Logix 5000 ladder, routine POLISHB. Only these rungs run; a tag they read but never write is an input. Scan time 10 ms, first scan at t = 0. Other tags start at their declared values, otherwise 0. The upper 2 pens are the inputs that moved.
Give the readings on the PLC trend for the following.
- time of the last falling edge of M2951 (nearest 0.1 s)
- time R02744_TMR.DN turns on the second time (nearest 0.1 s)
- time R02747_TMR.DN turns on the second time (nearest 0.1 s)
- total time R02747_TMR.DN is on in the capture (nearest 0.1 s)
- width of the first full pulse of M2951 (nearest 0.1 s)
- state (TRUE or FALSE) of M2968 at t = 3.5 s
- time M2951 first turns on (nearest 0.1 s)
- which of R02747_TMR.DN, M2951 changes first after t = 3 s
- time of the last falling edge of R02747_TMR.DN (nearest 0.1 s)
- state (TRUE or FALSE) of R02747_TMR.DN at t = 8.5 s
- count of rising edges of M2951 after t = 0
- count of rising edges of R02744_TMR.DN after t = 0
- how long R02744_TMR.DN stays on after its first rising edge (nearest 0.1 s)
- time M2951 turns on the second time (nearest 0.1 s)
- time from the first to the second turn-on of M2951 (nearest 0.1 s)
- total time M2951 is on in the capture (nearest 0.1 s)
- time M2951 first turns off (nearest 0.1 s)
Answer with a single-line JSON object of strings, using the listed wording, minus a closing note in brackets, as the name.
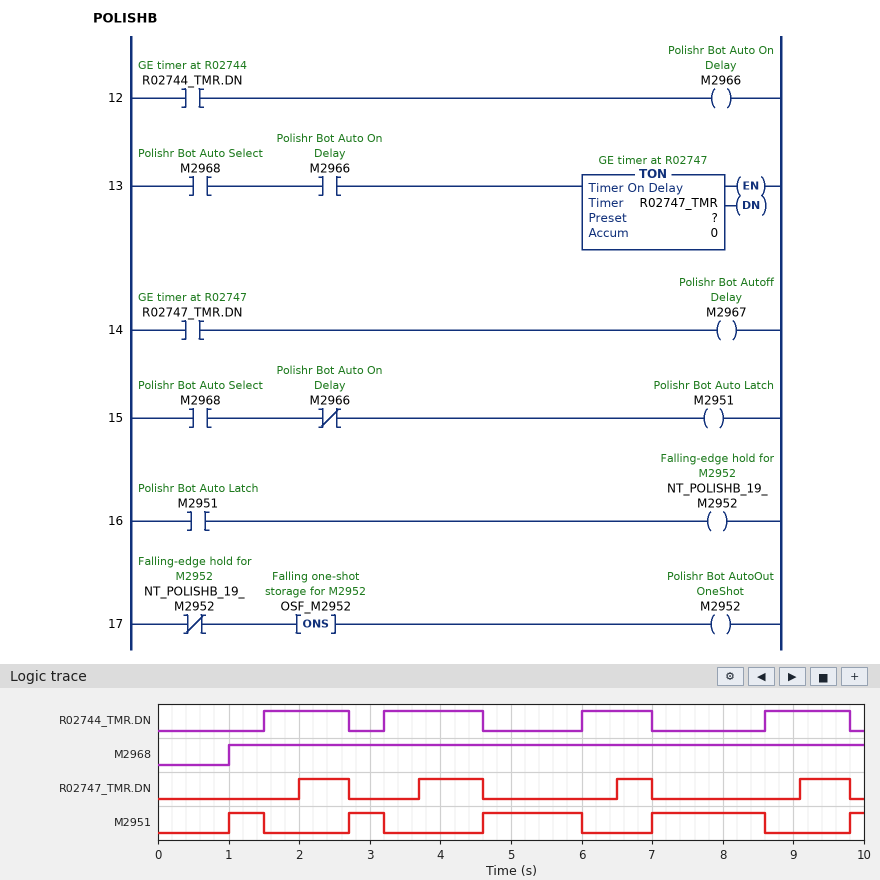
{"time of the last falling edge of M2951": "8.6 s", "time R02744_TMR.DN turns on the second time": "3.2 s", "time R02747_TMR.DN turns on the second time": "3.7 s", "total time R02747_TMR.DN is on in the capture": "2.8 s", "width of the first full pulse of M2951": "0.5 s", "state (TRUE or FALSE) of M2968 at t = 3.5 s": "TRUE", "time M2951 first turns on": "1.0 s", "which of R02747_TMR.DN, M2951 changes first after t = 3 s": "M2951", "time of the last falling edge of R02747_TMR.DN": "9.8 s", "state (TRUE or FALSE) of R02747_TMR.DN at t = 8.5 s": "FALSE", "count of rising edges of M2951 after t = 0": "5", "count of rising edges of R02744_TMR.DN after t = 0": "4", "how long R02744_TMR.DN stays on after its first rising edge": "1.2 s", "time M2951 turns on the second time": "2.7 s", "time from the first to the second turn-on of M2951": "1.7 s", "total time M2951 is on in the capture": "4.2 s", "time M2951 first turns off": "1.5 s"}
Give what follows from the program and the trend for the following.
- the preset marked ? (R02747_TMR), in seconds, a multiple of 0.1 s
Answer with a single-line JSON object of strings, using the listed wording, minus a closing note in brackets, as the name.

{"the preset marked ? (R02747_TMR), in seconds, a multiple of 0.1 s": "0.5 s"}
